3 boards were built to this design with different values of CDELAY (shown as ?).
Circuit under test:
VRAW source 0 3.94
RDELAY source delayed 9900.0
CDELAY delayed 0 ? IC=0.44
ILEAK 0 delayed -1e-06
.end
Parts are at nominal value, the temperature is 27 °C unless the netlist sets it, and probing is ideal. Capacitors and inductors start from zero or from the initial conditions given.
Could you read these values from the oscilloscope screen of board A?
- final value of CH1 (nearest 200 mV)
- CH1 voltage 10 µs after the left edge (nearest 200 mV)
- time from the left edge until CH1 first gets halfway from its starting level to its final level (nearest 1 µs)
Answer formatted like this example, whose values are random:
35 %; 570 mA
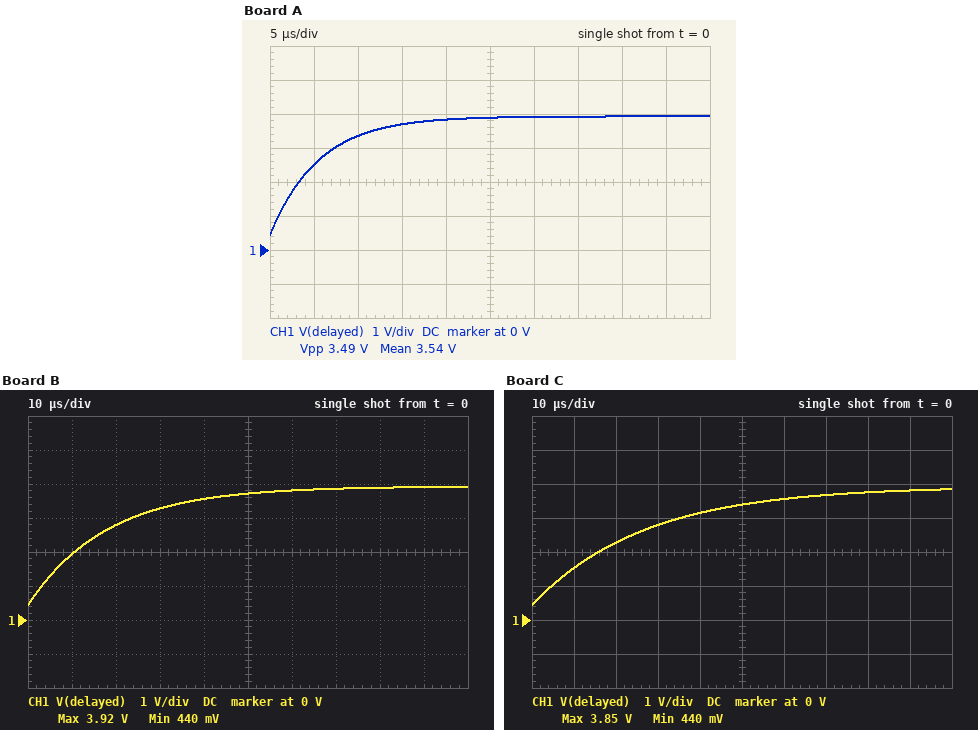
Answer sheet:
4.0 V; 3.4 V; 4 µs
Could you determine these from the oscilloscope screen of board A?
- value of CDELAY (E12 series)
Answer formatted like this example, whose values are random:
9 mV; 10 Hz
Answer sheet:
560 pF
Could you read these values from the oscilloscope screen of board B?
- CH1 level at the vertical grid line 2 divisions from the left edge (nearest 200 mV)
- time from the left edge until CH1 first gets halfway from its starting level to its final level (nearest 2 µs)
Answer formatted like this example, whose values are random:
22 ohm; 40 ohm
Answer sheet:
2.8 V; 12 µs
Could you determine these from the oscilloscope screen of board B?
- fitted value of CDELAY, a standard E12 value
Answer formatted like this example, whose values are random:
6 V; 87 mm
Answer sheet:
1.8 nF
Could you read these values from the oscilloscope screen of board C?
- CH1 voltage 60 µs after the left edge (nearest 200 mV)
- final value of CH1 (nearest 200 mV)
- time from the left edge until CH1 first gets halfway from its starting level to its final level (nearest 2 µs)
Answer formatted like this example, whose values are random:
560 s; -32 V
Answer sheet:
3.6 V; 3.8 V; 18 µs
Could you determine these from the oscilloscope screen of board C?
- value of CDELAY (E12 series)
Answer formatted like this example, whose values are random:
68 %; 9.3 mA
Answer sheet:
2.7 nF
